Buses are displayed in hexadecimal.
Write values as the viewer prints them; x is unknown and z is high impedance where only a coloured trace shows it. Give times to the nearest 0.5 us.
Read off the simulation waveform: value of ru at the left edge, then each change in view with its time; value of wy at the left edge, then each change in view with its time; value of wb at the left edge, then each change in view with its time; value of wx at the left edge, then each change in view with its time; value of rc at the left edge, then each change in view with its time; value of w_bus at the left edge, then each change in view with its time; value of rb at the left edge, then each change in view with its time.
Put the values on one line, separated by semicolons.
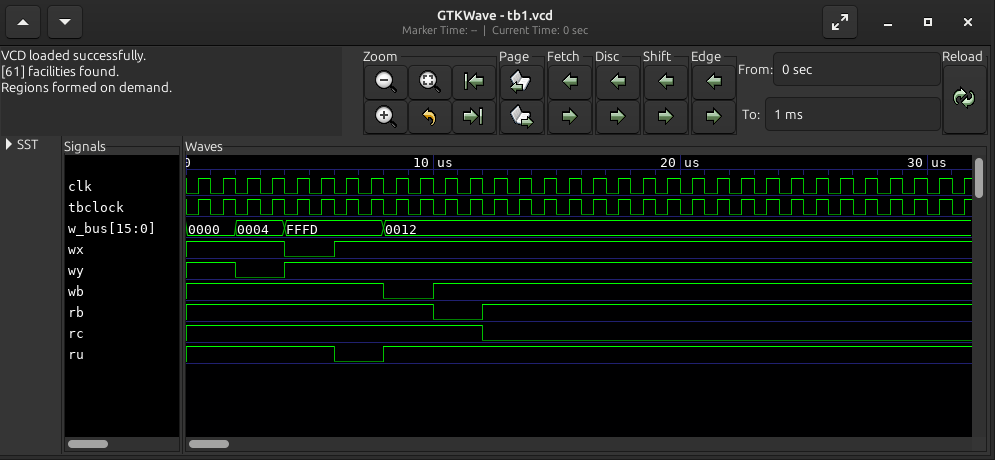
1, 0 at 6 us, 1 at 8 us; 1, 0 at 2 us, 1 at 4 us; 1, 0 at 8 us, 1 at 10 us; 1, 0 at 4 us, 1 at 6 us; 1, 0 at 12 us; 0000, 0004 at 2 us, FFFD at 4 us, 0012 at 8 us; 1, 0 at 10 us, 1 at 12 us
